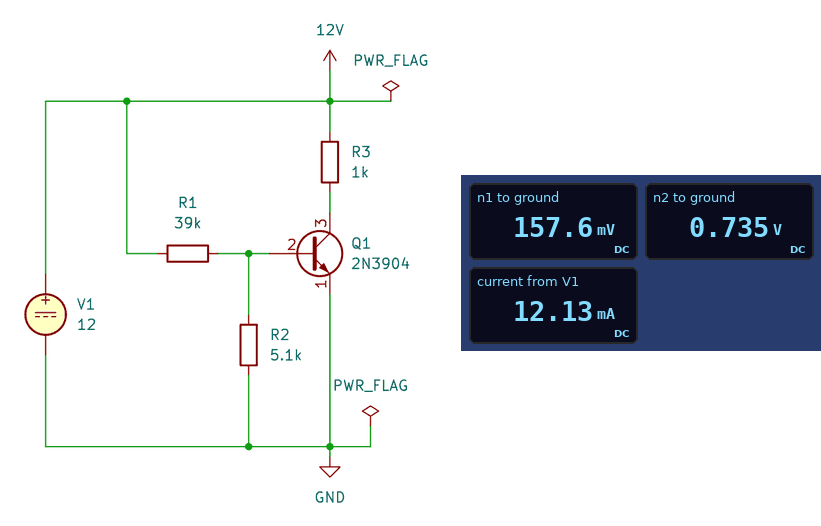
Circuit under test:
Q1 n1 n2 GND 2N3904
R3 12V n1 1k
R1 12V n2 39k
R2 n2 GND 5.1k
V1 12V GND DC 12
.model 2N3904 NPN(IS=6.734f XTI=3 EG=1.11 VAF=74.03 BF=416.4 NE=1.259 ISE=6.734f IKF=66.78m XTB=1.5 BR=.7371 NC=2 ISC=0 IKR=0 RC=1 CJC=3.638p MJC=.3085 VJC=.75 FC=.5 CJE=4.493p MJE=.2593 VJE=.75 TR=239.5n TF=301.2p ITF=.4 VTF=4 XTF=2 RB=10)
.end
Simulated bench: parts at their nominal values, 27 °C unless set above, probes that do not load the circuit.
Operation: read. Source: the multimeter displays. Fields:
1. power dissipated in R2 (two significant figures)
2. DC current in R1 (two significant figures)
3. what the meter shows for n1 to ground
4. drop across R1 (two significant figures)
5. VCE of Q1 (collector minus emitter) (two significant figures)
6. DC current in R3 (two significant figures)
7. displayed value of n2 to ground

110 µW
290 µA
157.6 mV
11 V
160 mV
12 mA
0.735 V
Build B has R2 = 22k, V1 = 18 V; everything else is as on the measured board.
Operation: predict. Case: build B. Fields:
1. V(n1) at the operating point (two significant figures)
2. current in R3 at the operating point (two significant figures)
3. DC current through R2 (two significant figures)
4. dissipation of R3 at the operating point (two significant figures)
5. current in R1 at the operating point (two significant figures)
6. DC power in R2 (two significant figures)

140 mV
18 mA
34 µA
320 mW
440 µA
26 µW
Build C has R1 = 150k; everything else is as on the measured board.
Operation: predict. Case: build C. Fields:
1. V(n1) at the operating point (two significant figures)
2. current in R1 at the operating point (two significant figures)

12 V
77 µA
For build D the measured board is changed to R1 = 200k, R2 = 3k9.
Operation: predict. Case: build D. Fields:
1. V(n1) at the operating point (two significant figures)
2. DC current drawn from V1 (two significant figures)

12 V
59 µA
